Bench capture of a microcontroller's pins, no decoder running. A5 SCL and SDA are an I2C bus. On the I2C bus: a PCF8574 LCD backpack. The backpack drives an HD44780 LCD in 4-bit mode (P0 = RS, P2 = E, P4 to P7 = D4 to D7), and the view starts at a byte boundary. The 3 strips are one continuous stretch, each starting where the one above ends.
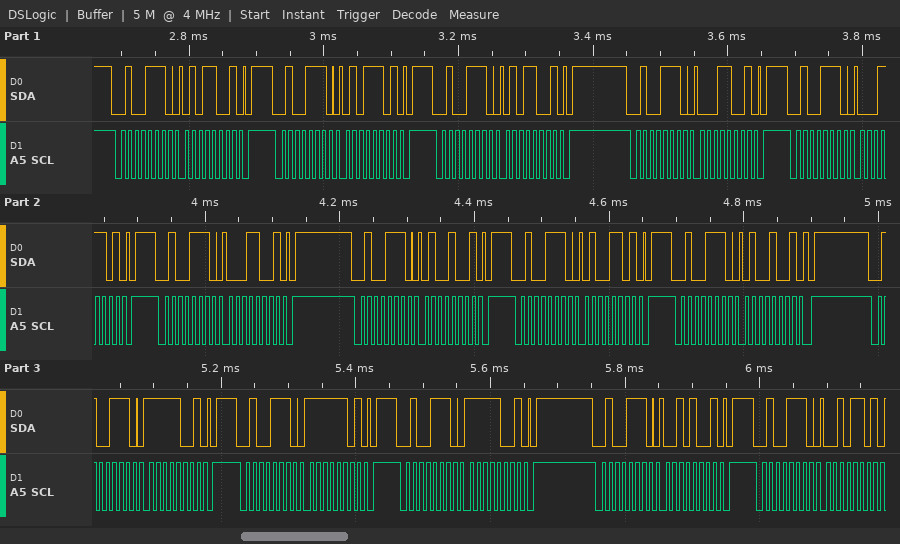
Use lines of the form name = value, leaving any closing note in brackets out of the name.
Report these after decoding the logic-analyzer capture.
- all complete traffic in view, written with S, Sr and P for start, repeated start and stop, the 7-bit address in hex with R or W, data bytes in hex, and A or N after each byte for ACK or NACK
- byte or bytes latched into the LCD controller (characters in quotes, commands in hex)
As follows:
all complete traffic in view, written with S, Sr and P for start, repeated start and stop, the 7-bit address in hex with R or W, data bytes in hex, and A or N after each byte for ACK or NACK = S 27W A 59 A P S 27W A 5D A P S 27W A 59 A P S 27W A 19 A P S 27W A 1D A P S 27W A 19 A P S 27W A 49 A P S 27W A 4D A P S 27W A 49 A P S 27W A F9 A P S 27W A FD A P S 27W A F9 A P S 27W A 29 A P S 27W A 2D A
byte or bytes latched into the LCD controller = 'Q' 'O'
